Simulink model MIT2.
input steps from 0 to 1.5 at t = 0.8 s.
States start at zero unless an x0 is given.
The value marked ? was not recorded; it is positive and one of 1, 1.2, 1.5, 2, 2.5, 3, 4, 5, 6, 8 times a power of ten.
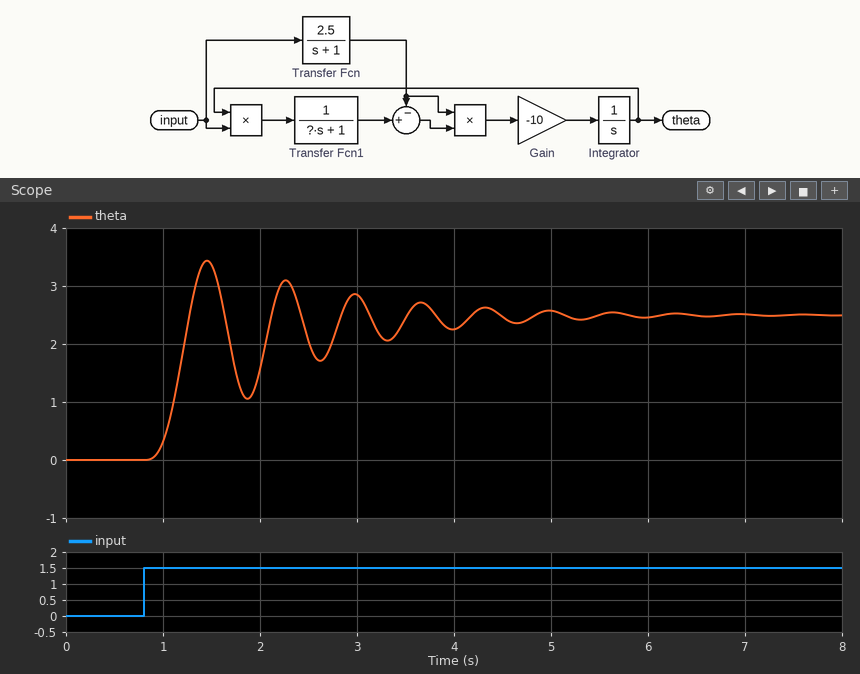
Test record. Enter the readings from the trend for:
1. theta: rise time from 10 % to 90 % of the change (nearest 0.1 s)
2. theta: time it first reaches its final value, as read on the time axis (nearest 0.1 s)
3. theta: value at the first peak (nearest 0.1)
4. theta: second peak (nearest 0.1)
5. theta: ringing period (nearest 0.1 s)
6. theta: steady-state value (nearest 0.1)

0.3 s
1.3 s
3.4
3.1
0.8 s
2.5
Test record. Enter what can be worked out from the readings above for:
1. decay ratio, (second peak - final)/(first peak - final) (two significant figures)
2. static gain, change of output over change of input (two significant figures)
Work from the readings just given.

0.67
1.7
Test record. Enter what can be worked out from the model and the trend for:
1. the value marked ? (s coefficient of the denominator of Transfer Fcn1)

0.6
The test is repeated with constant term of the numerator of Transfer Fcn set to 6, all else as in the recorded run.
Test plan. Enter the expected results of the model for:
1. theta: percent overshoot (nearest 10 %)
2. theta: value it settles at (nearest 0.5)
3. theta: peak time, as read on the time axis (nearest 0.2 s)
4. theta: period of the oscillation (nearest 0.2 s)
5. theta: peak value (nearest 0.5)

40 %
6.0
1.2 s
0.6 s
8.5
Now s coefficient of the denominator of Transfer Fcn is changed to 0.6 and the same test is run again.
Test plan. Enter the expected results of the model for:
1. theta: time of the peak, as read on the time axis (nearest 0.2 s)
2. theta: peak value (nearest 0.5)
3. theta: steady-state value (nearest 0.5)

1.4 s
5.0
2.5
